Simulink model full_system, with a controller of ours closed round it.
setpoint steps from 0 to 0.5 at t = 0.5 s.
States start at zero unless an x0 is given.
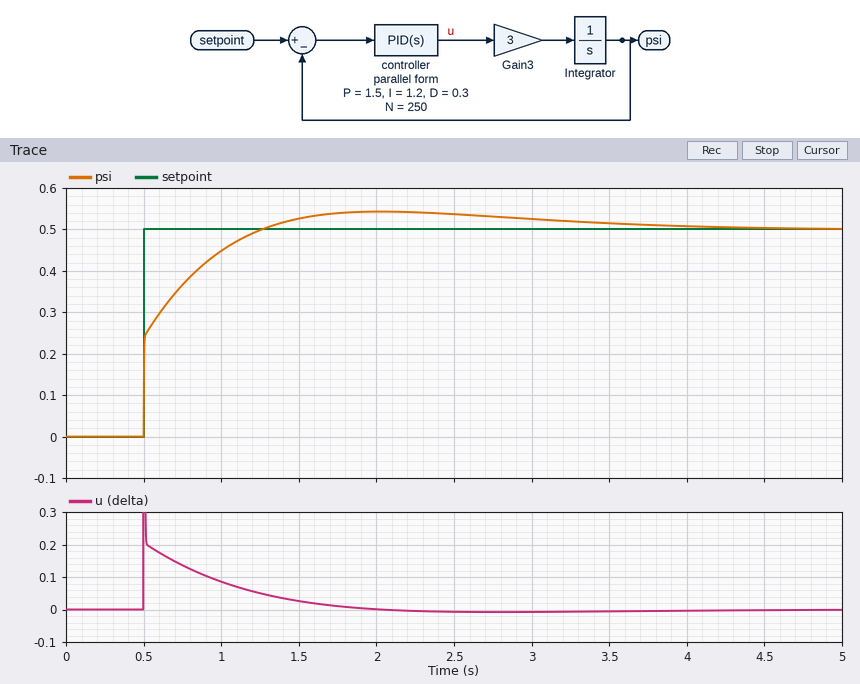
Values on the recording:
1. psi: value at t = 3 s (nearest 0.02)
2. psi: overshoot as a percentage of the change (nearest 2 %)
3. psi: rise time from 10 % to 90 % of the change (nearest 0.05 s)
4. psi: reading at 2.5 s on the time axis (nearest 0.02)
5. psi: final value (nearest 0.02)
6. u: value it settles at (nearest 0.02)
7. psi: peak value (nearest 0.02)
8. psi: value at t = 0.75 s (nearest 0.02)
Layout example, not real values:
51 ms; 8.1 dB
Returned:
0.52; 8 %; 0.50 s; 0.54; 0.50; 0.00; 0.54; 0.36
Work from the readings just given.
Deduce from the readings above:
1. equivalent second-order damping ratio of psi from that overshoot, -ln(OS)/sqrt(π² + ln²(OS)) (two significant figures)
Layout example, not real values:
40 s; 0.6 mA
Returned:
0.63
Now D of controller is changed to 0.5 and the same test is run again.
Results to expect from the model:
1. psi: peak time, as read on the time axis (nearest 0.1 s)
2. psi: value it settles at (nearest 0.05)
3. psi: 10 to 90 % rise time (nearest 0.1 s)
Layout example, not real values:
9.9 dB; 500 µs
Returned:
2.3 s; 0.50; 0.6 s
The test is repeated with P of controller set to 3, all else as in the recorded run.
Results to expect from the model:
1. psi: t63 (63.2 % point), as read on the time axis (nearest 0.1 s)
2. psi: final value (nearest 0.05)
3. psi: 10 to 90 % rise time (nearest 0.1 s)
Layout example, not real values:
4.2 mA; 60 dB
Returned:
0.6 s; 0.50; 0.3 s
